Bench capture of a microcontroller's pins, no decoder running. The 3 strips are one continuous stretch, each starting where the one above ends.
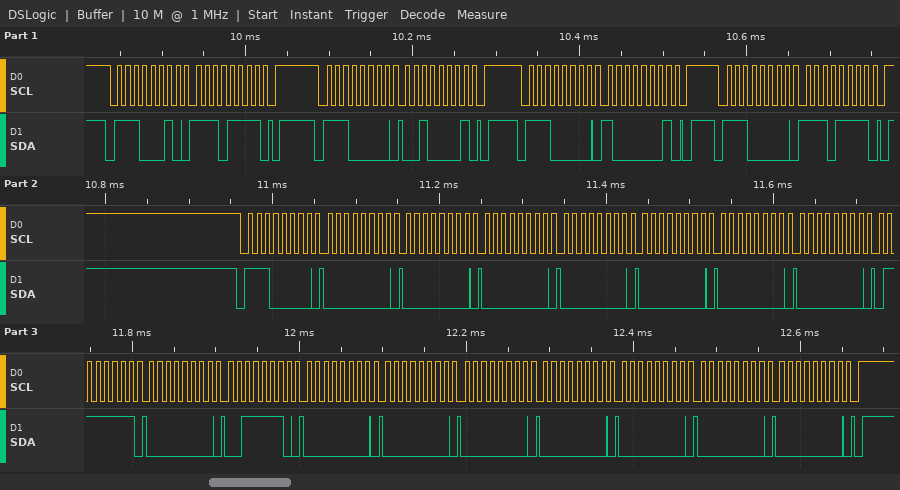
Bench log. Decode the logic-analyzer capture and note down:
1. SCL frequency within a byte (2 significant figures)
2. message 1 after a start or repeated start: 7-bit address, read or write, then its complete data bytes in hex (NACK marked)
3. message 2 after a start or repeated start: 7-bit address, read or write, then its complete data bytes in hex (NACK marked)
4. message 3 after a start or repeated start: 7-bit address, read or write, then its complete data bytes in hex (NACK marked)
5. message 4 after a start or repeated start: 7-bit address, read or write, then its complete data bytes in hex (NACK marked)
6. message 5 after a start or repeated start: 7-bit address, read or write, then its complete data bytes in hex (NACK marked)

100 kHz
0x71 write: EF
0x70 write: 21
0x70 write: 81
0x70 write: EF
0x70 write: 00 00 00 00 00 00 00 7F 00 3E 00 00 00 00 00 00 00
